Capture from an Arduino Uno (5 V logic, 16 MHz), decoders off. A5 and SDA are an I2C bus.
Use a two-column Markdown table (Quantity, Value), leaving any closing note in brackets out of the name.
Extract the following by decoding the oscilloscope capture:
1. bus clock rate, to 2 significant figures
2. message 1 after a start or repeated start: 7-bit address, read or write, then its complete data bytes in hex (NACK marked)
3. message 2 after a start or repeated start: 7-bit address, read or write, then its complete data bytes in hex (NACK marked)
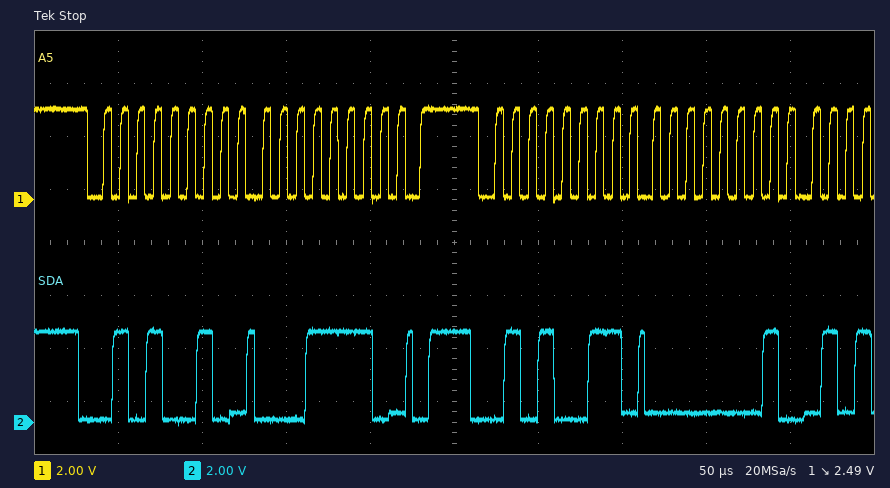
| Quantity | Value |
|---|---|
| bus clock rate, to 2 significant figures | 100 kHz |
| message 1 after a start or repeated start: 7-bit address, read or write, then its complete data bytes in hex | 0x29 write: 1E |
| message 2 after a start or repeated start: 7-bit address, read or write, then its complete data bytes in hex | 0x29 read: 01 |
